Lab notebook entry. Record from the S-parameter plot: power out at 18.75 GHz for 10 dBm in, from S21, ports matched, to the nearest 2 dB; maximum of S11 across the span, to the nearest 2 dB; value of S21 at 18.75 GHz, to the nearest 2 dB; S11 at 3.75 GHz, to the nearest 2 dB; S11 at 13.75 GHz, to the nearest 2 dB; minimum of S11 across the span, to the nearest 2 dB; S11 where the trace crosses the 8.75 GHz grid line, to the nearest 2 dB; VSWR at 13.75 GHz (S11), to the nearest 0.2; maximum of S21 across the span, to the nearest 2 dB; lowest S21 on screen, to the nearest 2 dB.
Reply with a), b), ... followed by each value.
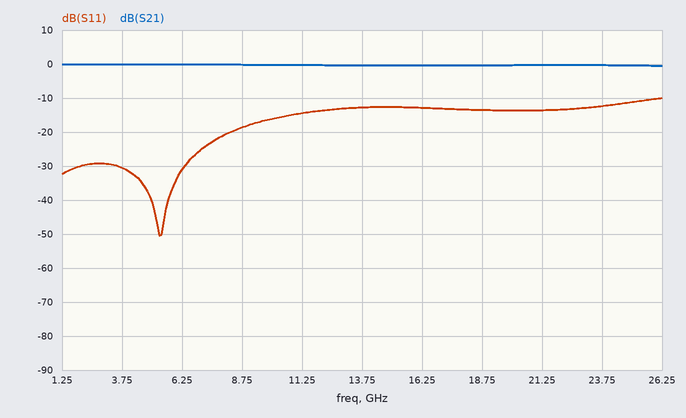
a) 10 dBm
b) -10 dB
c) 0 dB
d) -30 dB
e) -12 dB
f) -50 dB
g) -18 dB
h) 1.6
i) 0 dB
j) 0 dB
